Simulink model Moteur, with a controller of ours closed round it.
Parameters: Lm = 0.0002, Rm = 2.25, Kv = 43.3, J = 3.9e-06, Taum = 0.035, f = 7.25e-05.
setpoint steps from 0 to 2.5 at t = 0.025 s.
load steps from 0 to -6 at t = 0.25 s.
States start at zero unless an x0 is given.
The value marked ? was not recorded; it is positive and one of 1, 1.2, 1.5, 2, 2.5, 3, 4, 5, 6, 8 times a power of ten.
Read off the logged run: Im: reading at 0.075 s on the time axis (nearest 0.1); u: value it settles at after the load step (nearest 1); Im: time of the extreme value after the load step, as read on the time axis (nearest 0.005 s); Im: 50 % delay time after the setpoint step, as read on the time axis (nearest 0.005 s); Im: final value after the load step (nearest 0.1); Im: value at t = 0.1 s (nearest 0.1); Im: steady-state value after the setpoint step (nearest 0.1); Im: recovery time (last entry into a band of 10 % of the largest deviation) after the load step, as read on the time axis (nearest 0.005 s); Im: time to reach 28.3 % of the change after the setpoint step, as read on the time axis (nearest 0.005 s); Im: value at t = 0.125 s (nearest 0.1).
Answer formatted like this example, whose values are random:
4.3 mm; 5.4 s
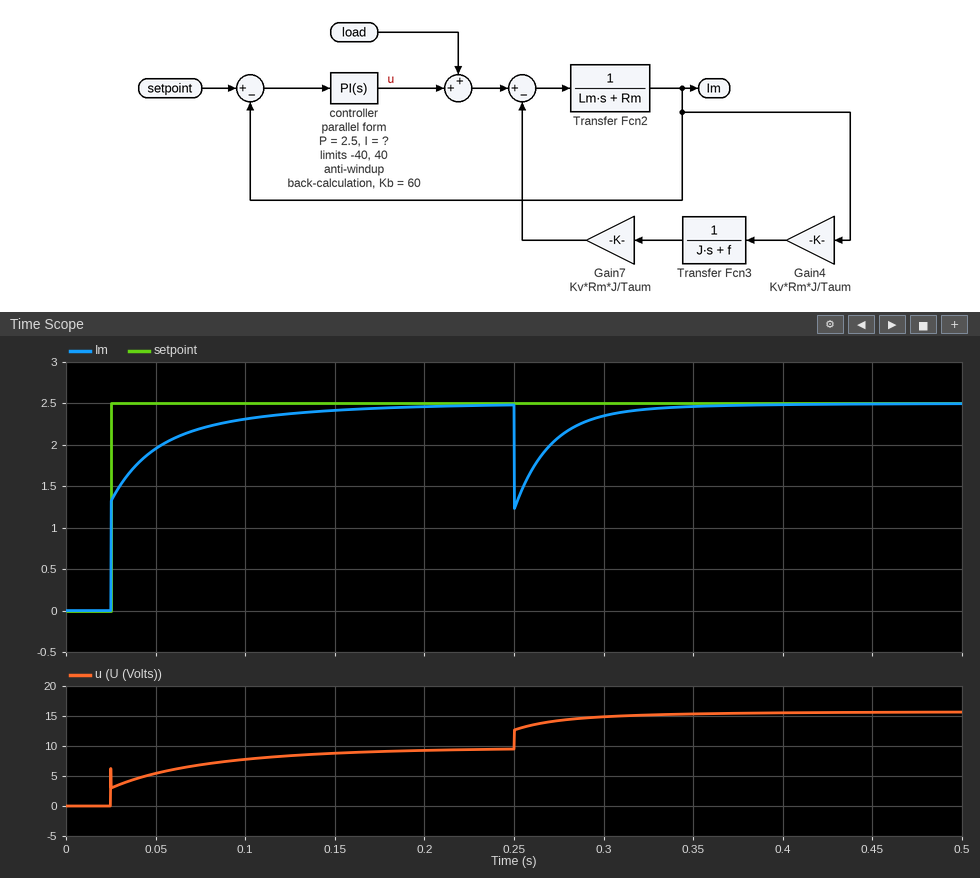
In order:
2.2; 16; 0.250 s; 0.025 s; 2.5; 2.3; 2.5; 0.305 s; 0.025 s; 2.4
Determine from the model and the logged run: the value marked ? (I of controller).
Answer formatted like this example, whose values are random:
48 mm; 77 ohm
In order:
200
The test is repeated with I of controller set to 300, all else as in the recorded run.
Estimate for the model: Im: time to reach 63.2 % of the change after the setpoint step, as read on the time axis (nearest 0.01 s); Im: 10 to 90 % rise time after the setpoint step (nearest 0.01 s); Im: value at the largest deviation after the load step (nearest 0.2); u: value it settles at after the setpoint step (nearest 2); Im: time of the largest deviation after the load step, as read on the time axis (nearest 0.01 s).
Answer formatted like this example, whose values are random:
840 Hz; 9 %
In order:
0.03 s; 0.04 s; 1.2; 10; 0.25 s
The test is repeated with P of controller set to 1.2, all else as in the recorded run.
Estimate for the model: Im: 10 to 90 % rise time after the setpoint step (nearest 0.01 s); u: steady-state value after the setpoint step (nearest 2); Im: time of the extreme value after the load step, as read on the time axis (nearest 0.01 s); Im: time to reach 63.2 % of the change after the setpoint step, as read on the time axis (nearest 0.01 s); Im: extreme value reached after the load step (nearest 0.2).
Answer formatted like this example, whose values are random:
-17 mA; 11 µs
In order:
0.05 s; 10; 0.25 s; 0.04 s; 0.8
